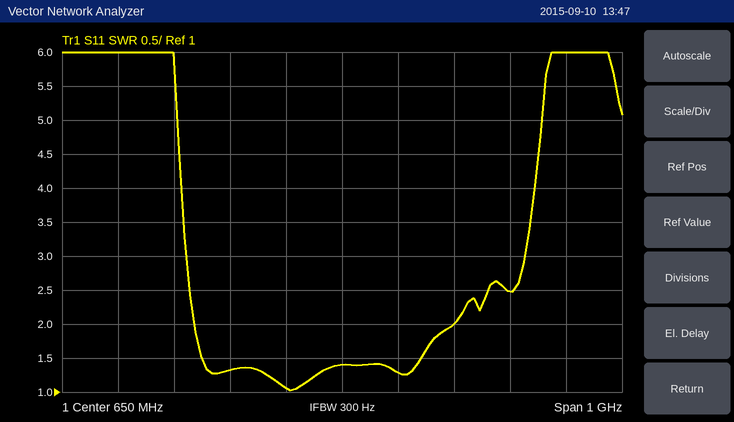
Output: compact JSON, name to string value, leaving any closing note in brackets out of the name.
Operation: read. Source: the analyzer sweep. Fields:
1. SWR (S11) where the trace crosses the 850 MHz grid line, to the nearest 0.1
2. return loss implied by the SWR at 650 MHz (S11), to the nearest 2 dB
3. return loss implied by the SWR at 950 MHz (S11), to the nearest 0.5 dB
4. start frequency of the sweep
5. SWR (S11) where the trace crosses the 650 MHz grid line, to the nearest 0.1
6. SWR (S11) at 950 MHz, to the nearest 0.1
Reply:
{"SWR (S11) where the trace crosses the 850 MHz grid line, to the nearest 0.1": "2.0", "return loss implied by the SWR at 650 MHz (S11), to the nearest 2 dB": "16 dB", "return loss implied by the SWR at 950 MHz (S11), to the nearest 0.5 dB": "7.5 dB", "start frequency of the sweep": "150 MHz", "SWR (S11) where the trace crosses the 650 MHz grid line, to the nearest 0.1": "1.4", "SWR (S11) at 950 MHz, to the nearest 0.1": "2.5"}
